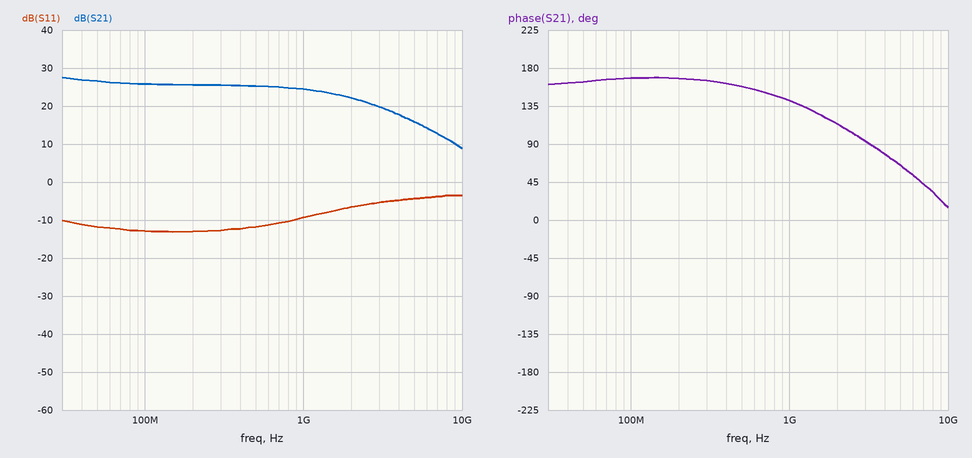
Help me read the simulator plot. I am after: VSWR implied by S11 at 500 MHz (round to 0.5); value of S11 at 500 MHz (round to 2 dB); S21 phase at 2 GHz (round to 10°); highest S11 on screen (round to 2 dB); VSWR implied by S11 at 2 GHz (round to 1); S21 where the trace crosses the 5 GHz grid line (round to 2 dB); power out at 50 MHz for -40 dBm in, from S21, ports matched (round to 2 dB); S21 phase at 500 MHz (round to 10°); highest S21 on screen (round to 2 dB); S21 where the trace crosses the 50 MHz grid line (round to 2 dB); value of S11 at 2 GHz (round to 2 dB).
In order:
1.5
-12 dB
110°
-4 dB
3
16 dB
-14 dBm
160°
28 dB
26 dB
-6 dB
